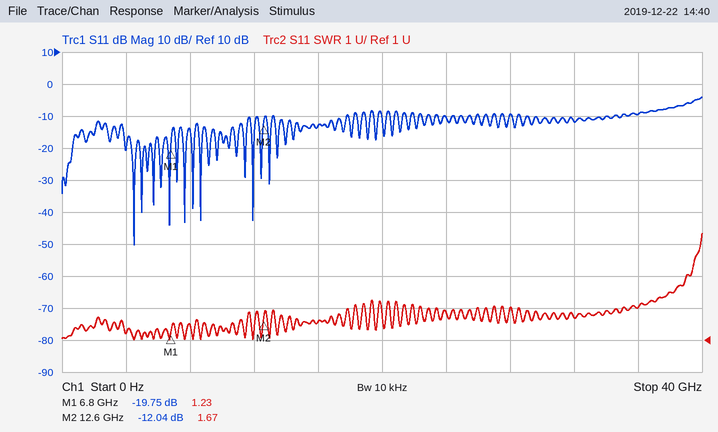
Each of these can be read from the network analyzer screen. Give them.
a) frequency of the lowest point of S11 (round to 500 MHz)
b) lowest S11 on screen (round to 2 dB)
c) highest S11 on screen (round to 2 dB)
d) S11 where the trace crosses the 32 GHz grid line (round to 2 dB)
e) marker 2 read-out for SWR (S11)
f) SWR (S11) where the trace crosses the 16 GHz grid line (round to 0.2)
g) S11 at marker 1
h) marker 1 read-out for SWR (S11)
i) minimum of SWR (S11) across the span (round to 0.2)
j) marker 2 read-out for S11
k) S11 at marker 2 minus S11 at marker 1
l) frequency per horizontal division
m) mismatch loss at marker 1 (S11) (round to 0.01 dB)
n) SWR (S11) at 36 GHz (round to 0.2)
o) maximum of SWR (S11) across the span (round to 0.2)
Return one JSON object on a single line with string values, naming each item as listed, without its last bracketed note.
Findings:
{"frequency of the lowest point of S11": "4.5 GHz", "lowest S11 on screen": "-50 dB", "highest S11 on screen": "-4 dB", "S11 where the trace crosses the 32 GHz grid line": "-12 dB", "marker 2 read-out for SWR": "1.67", "SWR (S11) where the trace crosses the 16 GHz grid line": "1.6", "S11 at marker 1": "-19.75 dB", "marker 1 read-out for SWR": "1.23", "minimum of SWR (S11) across the span": "1.0", "marker 2 read-out for S11": "-12.04 dB", "S11 at marker 2 minus S11 at marker 1": "7.71 dB", "frequency per horizontal division": "4 GHz", "mismatch loss at marker 1 (S11)": "0.05 dB", "SWR (S11) at 36 GHz": "2.0", "maximum of SWR (S11) across the span": "4.4"}
